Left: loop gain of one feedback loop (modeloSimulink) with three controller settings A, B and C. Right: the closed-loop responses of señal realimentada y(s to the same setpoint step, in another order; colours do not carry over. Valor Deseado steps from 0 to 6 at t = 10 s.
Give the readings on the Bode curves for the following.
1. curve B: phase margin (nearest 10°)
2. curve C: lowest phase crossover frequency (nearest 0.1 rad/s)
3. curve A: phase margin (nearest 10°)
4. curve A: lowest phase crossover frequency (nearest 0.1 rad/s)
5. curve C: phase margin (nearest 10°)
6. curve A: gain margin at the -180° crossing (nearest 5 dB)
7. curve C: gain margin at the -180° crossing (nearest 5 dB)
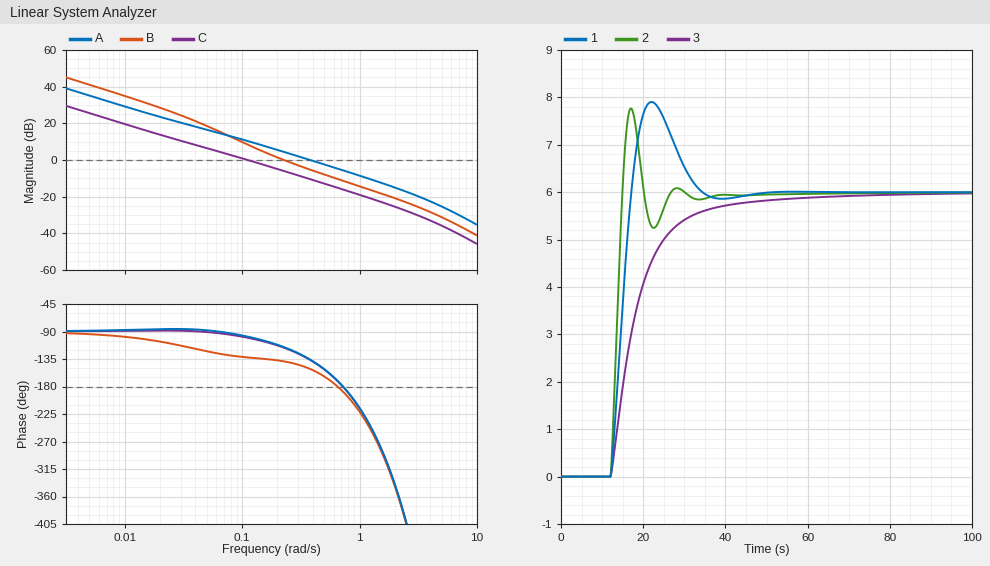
40°
0.7 rad/s
40°
0.7 rad/s
80°
5 dB
15 dB
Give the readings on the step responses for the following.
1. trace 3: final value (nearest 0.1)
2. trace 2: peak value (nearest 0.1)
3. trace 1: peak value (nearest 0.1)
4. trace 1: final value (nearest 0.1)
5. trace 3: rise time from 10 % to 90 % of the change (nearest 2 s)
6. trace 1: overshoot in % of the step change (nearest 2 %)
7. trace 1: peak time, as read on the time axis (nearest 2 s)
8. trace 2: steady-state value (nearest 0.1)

6.0
7.8
7.9
6.0
16 s
32 %
22 s
6.0
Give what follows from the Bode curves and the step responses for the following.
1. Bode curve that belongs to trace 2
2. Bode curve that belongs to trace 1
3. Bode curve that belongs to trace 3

A
B
C
